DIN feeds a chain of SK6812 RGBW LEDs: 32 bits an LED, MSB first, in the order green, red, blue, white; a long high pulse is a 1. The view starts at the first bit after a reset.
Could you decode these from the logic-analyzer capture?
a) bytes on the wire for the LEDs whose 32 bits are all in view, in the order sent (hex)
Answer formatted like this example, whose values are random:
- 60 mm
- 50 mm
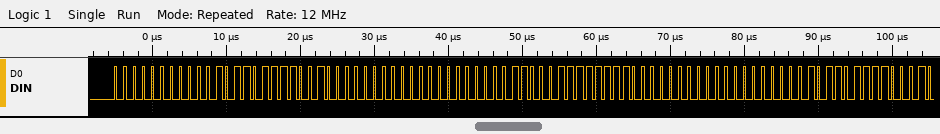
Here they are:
- 00 16 F2 00 00 18 FF 00
